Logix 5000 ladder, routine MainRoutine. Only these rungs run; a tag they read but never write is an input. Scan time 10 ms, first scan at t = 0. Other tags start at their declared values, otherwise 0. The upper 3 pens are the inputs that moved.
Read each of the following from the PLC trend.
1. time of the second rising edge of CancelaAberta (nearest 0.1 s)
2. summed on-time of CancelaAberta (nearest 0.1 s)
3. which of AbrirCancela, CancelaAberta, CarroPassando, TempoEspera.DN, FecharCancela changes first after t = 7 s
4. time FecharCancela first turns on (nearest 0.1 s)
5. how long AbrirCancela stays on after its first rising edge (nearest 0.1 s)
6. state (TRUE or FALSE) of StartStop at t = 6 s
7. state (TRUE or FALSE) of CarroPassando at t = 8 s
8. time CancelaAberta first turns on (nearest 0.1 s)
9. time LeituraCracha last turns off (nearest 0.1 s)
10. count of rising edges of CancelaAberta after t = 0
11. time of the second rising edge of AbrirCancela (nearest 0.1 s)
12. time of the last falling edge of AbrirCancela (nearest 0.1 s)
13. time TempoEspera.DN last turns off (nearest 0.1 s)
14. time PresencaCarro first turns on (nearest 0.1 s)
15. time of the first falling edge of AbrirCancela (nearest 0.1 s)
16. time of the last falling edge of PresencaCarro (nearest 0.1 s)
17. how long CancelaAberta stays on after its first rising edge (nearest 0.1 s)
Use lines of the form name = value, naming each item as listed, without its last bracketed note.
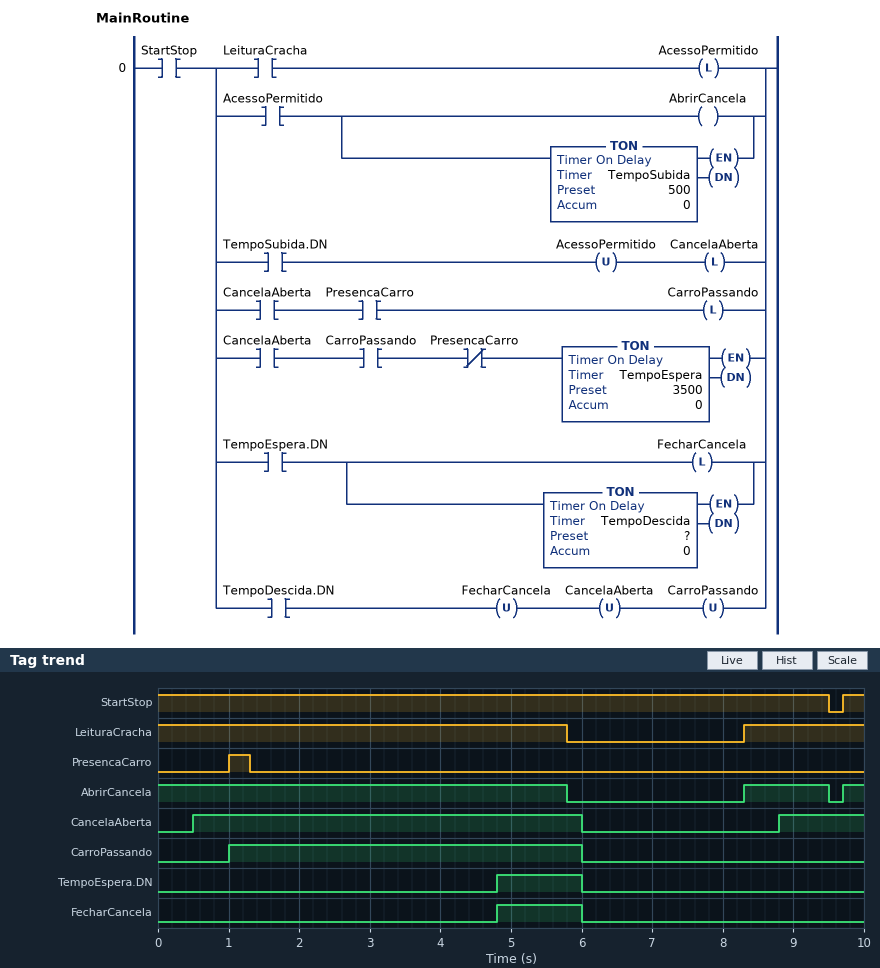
time of the second rising edge of CancelaAberta = 8.8 s
summed on-time of CancelaAberta = 6.7 s
which of AbrirCancela, CancelaAberta, CarroPassando, TempoEspera.DN, FecharCancela changes first after t = 7 s = AbrirCancela
time FecharCancela first turns on = 4.8 s
how long AbrirCancela stays on after its first rising edge = 1.2 s
state (TRUE or FALSE) of StartStop at t = 6 s = TRUE
state (TRUE or FALSE) of CarroPassando at t = 8 s = FALSE
time CancelaAberta first turns on = 0.5 s
time LeituraCracha last turns off = 5.8 s
count of rising edges of CancelaAberta after t = 0 = 2
time of the second rising edge of AbrirCancela = 9.7 s
time of the last falling edge of AbrirCancela = 9.5 s
time TempoEspera.DN last turns off = 6.0 s
time PresencaCarro first turns on = 1.0 s
time of the first falling edge of AbrirCancela = 5.8 s
time of the last falling edge of PresencaCarro = 1.3 s
how long CancelaAberta stays on after its first rising edge = 5.5 s
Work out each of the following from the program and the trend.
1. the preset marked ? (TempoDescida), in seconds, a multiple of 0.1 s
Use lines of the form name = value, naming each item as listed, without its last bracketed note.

the preset marked ? (TempoDescida), in seconds, a multiple of 0.1 s = 1.2 s
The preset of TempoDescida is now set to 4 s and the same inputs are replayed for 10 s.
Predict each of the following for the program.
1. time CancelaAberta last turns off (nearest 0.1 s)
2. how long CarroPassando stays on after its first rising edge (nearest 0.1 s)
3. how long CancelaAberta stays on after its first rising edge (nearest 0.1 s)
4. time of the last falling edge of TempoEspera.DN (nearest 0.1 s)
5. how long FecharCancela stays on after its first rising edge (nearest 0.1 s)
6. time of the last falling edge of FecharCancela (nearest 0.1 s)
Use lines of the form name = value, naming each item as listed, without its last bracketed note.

time CancelaAberta last turns off = 8.8 s
how long CarroPassando stays on after its first rising edge = 7.8 s
how long CancelaAberta stays on after its first rising edge = 8.3 s
time of the last falling edge of TempoEspera.DN = 8.8 s
how long FecharCancela stays on after its first rising edge = 4.0 s
time of the last falling edge of FecharCancela = 8.8 s
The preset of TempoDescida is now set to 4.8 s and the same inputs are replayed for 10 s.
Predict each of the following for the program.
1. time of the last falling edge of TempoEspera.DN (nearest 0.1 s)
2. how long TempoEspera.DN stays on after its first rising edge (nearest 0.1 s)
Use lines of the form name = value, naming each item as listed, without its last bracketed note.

time of the last falling edge of TempoEspera.DN = 9.5 s
how long TempoEspera.DN stays on after its first rising edge = 4.7 s
